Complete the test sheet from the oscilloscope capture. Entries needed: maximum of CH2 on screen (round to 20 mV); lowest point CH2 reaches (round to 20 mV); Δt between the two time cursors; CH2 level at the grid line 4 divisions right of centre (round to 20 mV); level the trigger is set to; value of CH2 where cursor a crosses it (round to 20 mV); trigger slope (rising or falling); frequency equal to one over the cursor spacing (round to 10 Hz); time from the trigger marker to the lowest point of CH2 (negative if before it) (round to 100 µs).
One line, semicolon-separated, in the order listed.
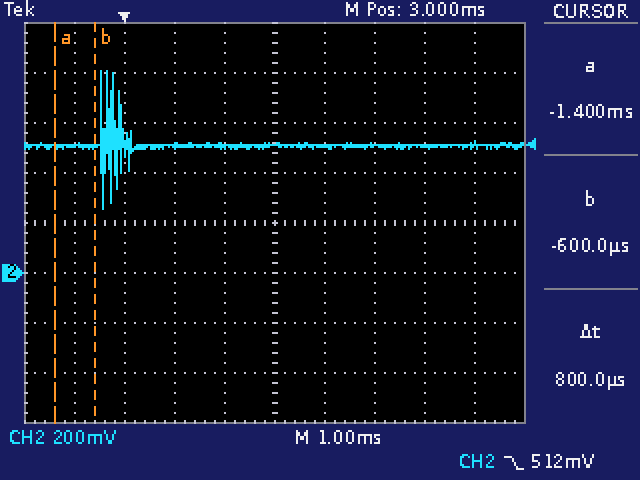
800 mV; 260 mV; 800 µs; 520 mV; 512 mV; 500 mV; falling; 1.25 kHz; -400 µs
